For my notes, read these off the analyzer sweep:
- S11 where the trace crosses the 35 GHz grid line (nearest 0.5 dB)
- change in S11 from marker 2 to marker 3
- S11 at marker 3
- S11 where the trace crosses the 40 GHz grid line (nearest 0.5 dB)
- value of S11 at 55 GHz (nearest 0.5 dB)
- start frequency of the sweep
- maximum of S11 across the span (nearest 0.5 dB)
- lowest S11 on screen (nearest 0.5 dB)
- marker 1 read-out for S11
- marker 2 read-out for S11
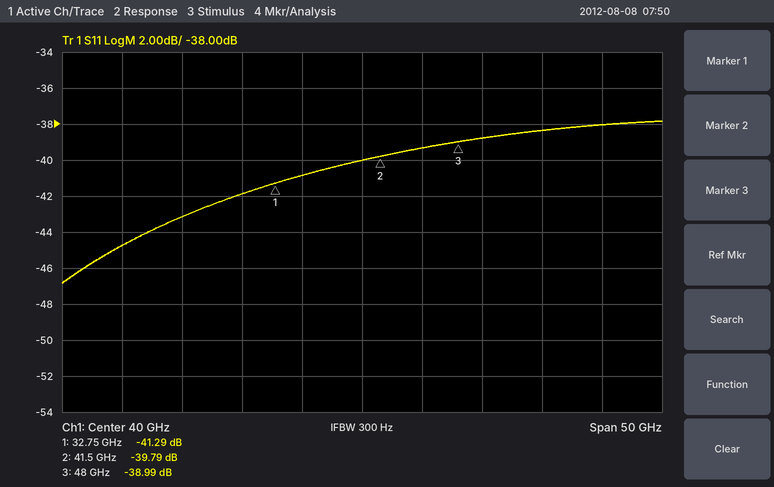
-41.0 dB
0.80 dB
-38.99 dB
-40.0 dB
-38.5 dB
15 GHz
-38.0 dB
-47.0 dB
-41.29 dB
-39.79 dB
